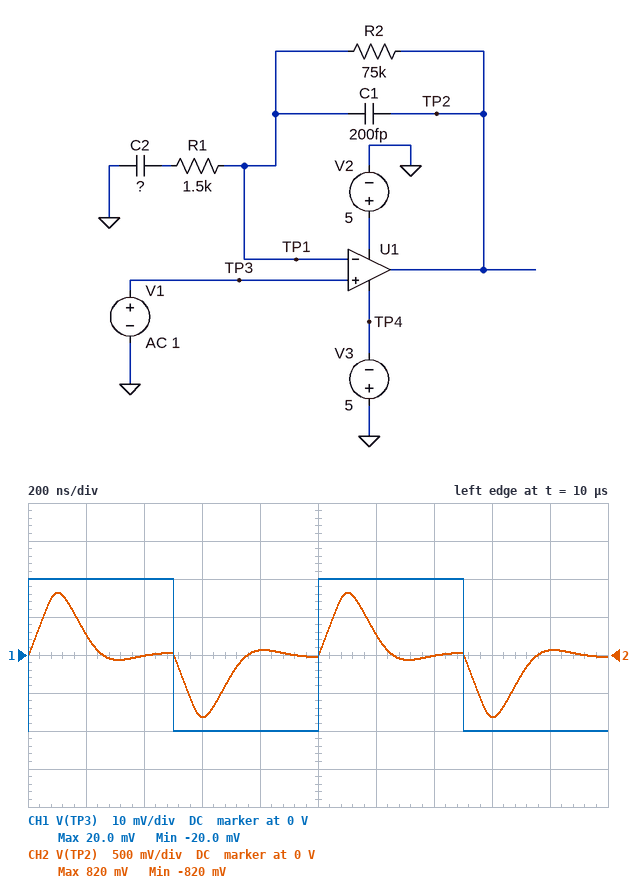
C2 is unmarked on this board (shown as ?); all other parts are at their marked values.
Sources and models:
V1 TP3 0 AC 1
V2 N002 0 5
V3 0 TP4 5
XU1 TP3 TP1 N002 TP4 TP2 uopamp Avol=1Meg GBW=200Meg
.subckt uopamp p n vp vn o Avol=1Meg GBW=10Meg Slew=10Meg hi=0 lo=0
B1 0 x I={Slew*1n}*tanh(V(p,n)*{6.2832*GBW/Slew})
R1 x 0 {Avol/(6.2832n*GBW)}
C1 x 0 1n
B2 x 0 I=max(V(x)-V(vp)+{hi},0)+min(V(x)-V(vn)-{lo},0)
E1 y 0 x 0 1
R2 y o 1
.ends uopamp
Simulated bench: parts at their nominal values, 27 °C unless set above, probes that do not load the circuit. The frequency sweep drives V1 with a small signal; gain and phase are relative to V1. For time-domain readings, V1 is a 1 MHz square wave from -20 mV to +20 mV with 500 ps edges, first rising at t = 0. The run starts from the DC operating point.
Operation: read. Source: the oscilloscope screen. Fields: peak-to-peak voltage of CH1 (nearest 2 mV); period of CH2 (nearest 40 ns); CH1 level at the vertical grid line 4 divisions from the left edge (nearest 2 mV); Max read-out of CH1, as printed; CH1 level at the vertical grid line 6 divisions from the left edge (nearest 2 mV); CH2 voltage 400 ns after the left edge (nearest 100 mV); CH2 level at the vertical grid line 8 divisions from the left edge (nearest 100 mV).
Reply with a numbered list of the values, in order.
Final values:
1. 40 mV
2. 1.00 µs
3. -20 mV
4. 20.0 mV
5. 20 mV
6. 0 V
7. -800 mV
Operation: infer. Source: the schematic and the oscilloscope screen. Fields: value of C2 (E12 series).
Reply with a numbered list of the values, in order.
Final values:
1. 33 pF
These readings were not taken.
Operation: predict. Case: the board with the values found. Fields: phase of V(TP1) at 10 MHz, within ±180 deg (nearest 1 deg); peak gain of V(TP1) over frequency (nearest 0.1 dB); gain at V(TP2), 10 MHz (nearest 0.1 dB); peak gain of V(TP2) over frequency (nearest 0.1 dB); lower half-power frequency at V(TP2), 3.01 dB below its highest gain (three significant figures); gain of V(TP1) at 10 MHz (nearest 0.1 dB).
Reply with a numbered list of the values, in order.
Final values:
1. -43 deg
2. 1.7 dB
3. 23.5 dB
4. 31.8 dB
5. 1.69 MHz
6. -7.5 dB
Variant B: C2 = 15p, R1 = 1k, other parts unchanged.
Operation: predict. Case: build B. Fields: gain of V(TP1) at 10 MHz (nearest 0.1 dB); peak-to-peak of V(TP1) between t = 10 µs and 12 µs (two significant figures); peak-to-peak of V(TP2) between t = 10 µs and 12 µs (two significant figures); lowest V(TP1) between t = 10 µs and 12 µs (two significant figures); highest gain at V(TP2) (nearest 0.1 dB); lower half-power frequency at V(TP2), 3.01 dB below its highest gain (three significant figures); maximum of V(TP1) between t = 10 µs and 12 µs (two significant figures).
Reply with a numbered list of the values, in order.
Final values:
1. -6.5 dB
2. 61 mV
3. 1.3 V
4. -31 mV
5. 31.5 dB
6. 3.04 MHz
7. 31 mV
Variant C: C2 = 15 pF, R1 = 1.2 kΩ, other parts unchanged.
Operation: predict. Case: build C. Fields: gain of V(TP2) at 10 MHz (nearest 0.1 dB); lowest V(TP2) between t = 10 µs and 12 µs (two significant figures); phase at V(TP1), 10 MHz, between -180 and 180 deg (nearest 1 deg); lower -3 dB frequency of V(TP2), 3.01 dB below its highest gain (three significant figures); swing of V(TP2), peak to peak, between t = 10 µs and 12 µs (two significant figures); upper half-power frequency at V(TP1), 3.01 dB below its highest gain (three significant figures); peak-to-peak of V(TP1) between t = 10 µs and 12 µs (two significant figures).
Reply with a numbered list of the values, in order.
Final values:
1. 24.7 dB
2. -620 mV
3. -59 deg
4. 2.89 MHz
5. 1.2 V
6. 6.09 MHz
7. 59 mV
